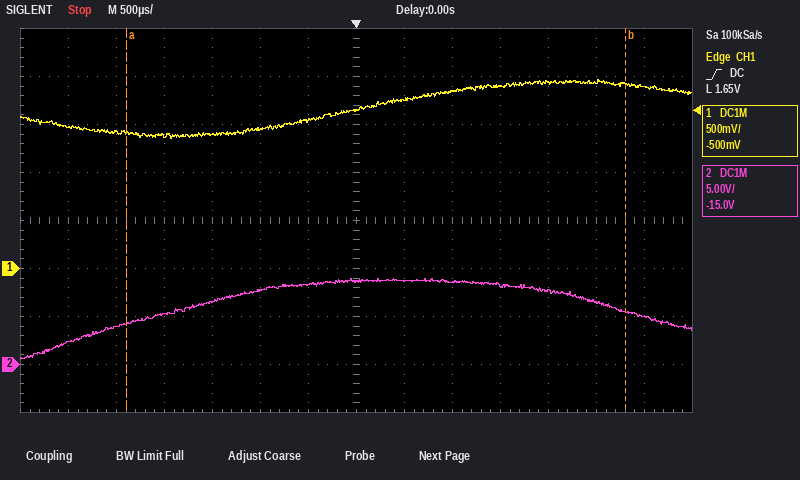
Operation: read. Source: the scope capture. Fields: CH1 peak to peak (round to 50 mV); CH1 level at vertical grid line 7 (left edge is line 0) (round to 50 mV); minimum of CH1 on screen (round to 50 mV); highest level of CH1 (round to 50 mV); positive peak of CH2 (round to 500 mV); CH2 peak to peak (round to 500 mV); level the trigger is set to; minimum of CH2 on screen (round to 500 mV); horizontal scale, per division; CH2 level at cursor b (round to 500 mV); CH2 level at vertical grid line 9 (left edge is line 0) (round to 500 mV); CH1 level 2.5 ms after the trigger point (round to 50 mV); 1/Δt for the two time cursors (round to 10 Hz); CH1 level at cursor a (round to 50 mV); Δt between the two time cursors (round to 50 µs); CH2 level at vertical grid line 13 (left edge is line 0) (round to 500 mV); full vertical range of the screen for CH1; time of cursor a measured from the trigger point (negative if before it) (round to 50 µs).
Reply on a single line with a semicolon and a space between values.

600 mV; 1.65 V; 1.35 V; 1.95 V; 9.0 V; 8.5 V; 1.65 V; 500 mV; 500 µs; 5.5 V; 8.5 V; 1.95 V; 190 Hz; 1.40 V; 5.20 ms; 5.0 V; 4 V; -2.40 ms
